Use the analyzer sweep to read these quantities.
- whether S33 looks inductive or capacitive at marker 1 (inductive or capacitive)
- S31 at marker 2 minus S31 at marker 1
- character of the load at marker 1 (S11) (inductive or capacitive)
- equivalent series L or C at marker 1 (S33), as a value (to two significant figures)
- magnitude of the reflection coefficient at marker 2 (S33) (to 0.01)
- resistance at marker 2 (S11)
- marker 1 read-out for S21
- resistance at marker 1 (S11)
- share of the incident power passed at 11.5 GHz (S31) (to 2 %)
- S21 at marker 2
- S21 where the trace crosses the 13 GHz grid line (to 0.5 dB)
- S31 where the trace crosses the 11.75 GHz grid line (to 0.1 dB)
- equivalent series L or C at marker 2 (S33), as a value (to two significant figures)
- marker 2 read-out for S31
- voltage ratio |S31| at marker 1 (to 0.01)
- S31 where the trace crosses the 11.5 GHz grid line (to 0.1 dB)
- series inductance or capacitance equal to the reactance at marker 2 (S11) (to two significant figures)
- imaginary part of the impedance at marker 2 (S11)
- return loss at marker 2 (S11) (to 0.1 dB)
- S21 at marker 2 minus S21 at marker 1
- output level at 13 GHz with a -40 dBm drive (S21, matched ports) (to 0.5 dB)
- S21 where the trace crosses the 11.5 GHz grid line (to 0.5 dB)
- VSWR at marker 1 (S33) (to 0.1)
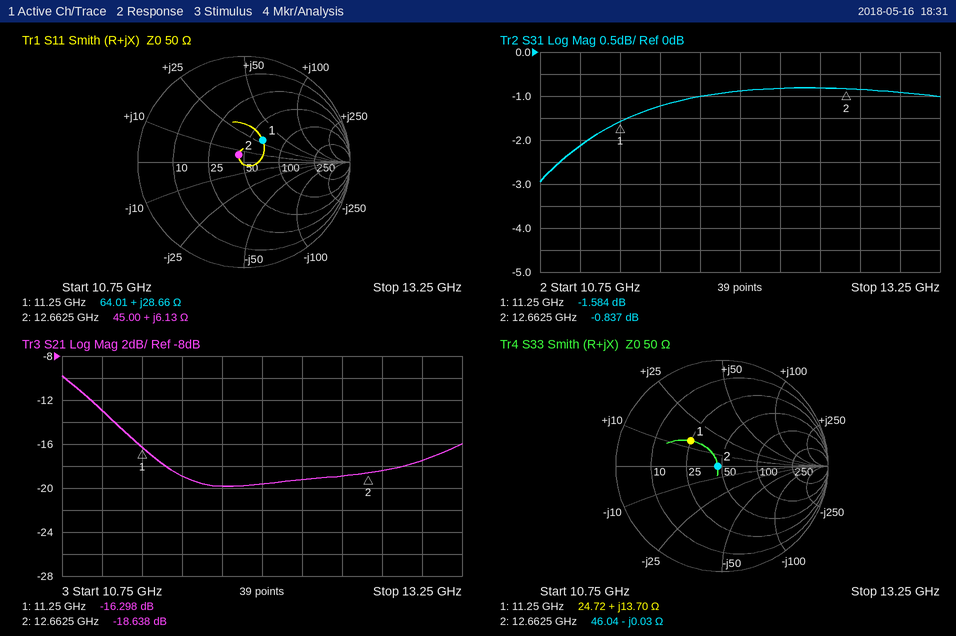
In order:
inductive
0.747 dB
inductive
190 pH
0.04
45.00 Ω
-16.298 dB
64.01 Ω
76 %
-18.638 dB
-17.5 dB
-1.0 dB
420 pF
-0.837 dB
0.83
-1.2 dB
77 pH
+6.13 Ω
21.6 dB
-2.340 dB
-57.5 dBm
-19.0 dB
2.2
